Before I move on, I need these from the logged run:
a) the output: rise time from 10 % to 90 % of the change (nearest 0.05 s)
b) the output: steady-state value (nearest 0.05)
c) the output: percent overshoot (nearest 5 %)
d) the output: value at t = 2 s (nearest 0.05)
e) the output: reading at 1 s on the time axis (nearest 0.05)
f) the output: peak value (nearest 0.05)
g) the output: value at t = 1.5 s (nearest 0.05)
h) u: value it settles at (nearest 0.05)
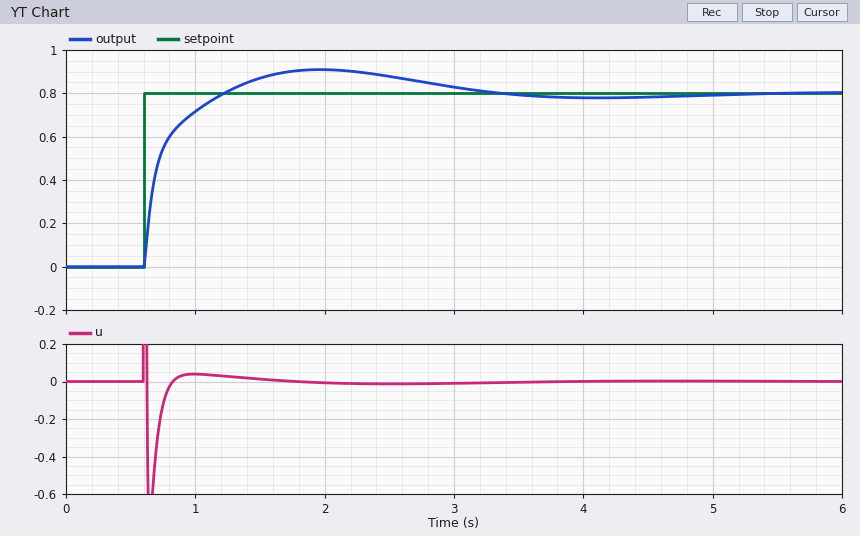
0.40 s
0.80
15 %
0.90
0.70
0.90
0.85
0.00
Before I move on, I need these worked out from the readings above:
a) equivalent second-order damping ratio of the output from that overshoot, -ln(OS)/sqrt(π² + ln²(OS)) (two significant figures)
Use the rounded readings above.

0.52
